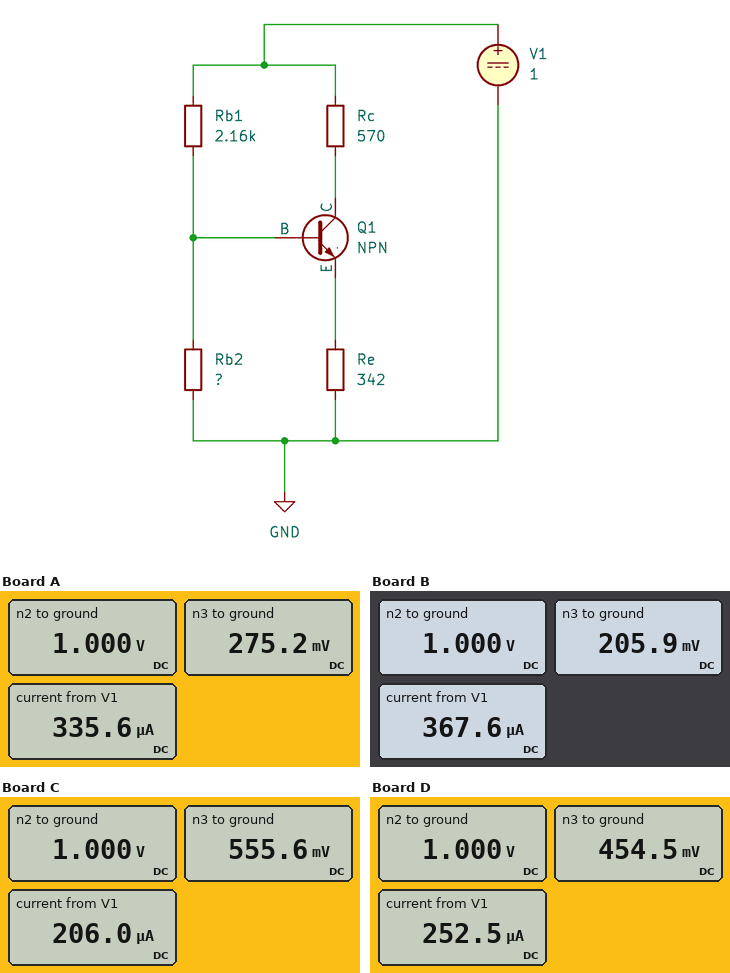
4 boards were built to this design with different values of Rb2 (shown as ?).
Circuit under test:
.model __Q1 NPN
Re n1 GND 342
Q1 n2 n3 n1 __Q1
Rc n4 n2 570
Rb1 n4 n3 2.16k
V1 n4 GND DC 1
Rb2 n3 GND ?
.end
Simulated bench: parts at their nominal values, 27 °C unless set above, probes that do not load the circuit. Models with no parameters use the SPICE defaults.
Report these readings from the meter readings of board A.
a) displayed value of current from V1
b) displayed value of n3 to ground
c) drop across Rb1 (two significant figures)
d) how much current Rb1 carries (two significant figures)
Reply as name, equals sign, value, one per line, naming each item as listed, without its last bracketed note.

displayed value of current from V1 = 335.6 µA
displayed value of n3 to ground = 275.2 mV
drop across Rb1 = 720 mV
how much current Rb1 carries = 340 µA
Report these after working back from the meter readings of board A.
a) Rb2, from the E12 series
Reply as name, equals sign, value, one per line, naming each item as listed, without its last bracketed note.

Rb2, from the E12 series = 820 Ω
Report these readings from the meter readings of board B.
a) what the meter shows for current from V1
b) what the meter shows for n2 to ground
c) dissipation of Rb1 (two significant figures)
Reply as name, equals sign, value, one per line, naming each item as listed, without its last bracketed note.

what the meter shows for current from V1 = 367.6 µA
what the meter shows for n2 to ground = 1.000 V
dissipation of Rb1 = 290 µW
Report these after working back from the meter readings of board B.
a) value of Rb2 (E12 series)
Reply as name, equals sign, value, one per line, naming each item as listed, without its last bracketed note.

value of Rb2 = 560 Ω
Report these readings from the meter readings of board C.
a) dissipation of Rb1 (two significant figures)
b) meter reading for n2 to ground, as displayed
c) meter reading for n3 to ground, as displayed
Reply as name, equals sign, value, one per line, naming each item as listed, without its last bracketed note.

dissipation of Rb1 = 91 µW
meter reading for n2 to ground, as displayed = 1.000 V
meter reading for n3 to ground, as displayed = 555.6 mV
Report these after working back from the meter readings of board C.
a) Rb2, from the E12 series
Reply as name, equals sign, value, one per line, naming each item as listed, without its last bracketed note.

Rb2, from the E12 series = 2.7 kΩ
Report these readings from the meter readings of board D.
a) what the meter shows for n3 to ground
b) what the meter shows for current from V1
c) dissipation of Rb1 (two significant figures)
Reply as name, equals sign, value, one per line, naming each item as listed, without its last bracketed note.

what the meter shows for n3 to ground = 454.5 mV
what the meter shows for current from V1 = 252.5 µA
dissipation of Rb1 = 140 µW
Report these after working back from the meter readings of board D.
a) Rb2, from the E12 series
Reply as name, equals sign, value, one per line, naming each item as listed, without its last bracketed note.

Rb2, from the E12 series = 1.8 kΩ
